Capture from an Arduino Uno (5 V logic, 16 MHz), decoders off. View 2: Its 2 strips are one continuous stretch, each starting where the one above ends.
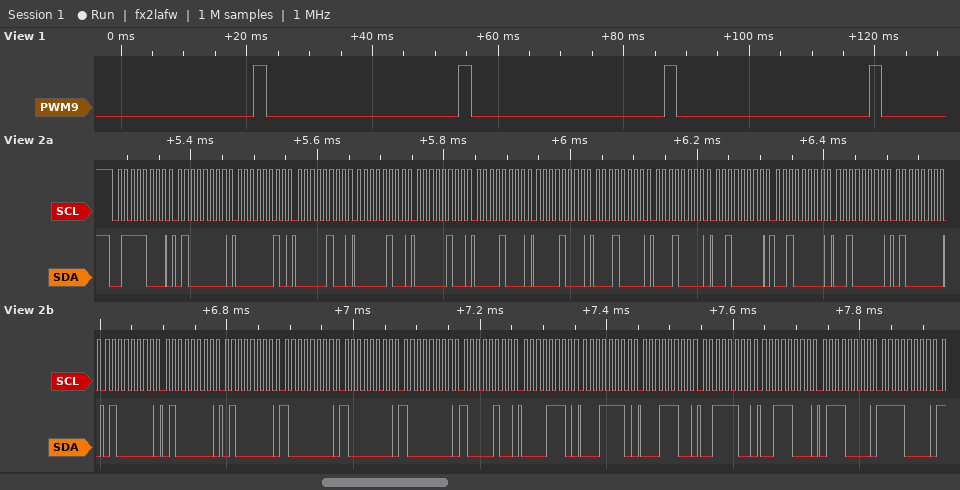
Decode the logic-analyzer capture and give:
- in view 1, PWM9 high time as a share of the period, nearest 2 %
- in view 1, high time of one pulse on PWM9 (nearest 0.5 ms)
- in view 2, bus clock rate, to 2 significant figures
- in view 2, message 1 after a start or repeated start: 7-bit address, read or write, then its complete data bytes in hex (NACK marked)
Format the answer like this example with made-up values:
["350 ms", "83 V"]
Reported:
["6 %", "2.0 ms", "100 kHz", "0x3C write: 40 02 04 04 04 08 08 10 10 20 20 20 40 40 40 40 80 80 80 84 0E 1E 1C 3C 38 70 F0"]
